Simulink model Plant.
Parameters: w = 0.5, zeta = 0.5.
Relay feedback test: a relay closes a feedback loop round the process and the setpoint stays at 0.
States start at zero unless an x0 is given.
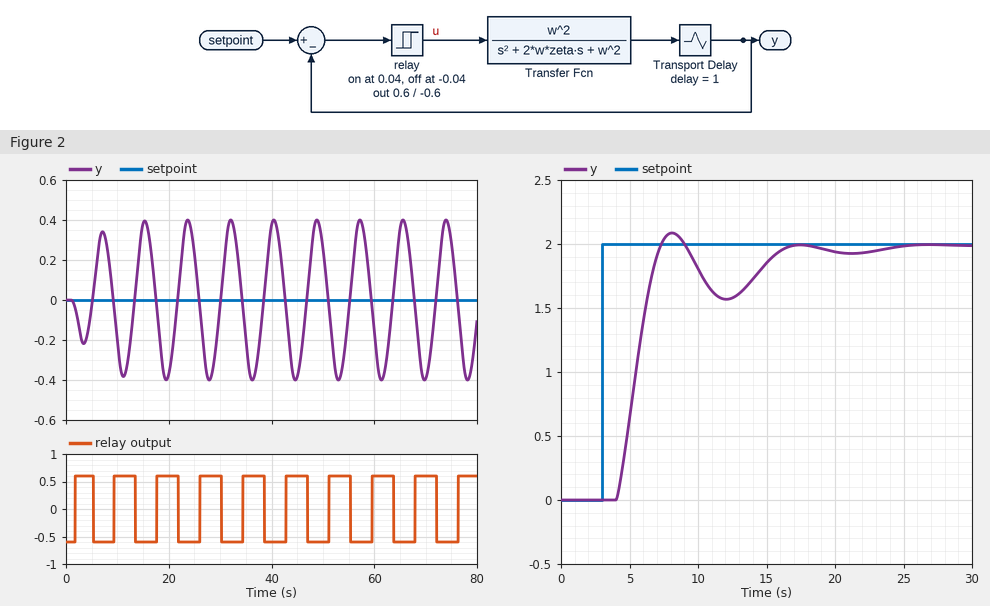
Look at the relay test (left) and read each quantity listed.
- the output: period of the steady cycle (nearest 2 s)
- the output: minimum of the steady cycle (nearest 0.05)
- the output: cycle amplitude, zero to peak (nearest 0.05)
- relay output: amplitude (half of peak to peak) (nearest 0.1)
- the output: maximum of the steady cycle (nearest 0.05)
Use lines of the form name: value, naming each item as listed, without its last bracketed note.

the output: period of the steady cycle: 8 s
the output: minimum of the steady cycle: -0.40
the output: cycle amplitude, zero to peak: 0.40
relay output: amplitude (half of peak to peak): 0.6
the output: maximum of the steady cycle: 0.40
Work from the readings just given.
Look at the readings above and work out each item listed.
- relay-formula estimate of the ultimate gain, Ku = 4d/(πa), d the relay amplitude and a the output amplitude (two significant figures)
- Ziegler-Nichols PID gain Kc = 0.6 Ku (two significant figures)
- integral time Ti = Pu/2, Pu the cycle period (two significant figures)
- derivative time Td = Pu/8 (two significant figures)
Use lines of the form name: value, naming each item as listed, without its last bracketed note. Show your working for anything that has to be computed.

relay-formula estimate of the ultimate gain, Ku = 4d/(πa), d the relay amplitude and a the output amplitude: 4 × 0.6 / (π × 0.4) = 1.9
Ziegler-Nichols PID gain Kc = 0.6 Ku: 0.6 × 1.9 = 1.1
integral time Ti = Pu/2, Pu the cycle period: 8 / 2 = 4.0 s
derivative time Td = Pu/8: 8 / 8 = 1.0 s
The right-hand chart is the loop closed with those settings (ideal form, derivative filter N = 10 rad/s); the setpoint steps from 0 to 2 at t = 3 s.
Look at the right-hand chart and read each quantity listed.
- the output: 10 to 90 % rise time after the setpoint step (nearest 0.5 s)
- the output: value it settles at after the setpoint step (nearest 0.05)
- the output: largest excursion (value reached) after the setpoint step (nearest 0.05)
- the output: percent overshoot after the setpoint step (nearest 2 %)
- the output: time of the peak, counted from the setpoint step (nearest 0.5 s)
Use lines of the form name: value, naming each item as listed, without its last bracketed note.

the output: 10 to 90 % rise time after the setpoint step: 2.5 s
the output: value it settles at after the setpoint step: 2.00
the output: largest excursion (value reached) after the setpoint step: 2.10
the output: percent overshoot after the setpoint step: 4 %
the output: time of the peak, counted from the setpoint step: 5.0 s
